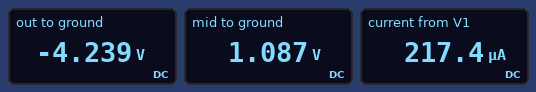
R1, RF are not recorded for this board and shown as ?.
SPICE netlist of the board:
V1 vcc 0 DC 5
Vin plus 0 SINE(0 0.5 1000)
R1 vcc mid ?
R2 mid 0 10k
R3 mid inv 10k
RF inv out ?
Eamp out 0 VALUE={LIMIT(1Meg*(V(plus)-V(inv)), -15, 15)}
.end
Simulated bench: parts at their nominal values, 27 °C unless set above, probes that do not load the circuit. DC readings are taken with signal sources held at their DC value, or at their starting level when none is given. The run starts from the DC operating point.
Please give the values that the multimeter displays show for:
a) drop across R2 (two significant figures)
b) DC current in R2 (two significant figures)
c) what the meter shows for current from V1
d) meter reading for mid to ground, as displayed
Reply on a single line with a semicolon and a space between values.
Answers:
1.1 V; 110 µA; 217.4 µA; 1.087 V
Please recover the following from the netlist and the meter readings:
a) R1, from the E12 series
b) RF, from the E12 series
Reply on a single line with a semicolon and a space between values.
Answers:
18 kΩ; 39 kΩ
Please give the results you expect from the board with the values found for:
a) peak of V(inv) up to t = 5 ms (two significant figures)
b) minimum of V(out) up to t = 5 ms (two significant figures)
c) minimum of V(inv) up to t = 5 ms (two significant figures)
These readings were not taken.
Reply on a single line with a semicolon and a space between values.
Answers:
500 mV; -5.9 V; -500 mV
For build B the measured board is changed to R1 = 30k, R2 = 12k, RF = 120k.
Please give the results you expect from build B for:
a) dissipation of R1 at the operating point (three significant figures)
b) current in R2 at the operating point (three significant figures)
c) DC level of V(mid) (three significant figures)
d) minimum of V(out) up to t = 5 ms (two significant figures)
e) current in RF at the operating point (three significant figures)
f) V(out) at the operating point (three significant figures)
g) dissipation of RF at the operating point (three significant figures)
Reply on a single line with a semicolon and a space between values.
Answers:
597 µW; 64.1 µA; 769 mV; -13 V; 76.9 µA; -9.23 V; 710 µW
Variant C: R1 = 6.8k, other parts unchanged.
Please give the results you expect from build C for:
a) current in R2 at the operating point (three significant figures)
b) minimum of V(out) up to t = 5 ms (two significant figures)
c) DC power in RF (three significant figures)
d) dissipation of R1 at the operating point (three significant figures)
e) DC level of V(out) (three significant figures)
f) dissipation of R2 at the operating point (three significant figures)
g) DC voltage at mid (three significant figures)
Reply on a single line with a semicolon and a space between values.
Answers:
212 µA; -10 V; 1.75 mW; 1.22 mW; -8.26 V; 449 µW; 2.12 V
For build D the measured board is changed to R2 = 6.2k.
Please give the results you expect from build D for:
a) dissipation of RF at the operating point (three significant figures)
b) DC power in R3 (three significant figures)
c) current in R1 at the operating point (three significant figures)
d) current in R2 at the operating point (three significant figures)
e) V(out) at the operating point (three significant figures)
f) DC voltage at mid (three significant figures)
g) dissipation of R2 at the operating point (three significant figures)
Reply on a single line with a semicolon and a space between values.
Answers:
300 µW; 76.9 µW; 229 µA; 141 µA; -3.42 V; 877 mV; 124 µW
